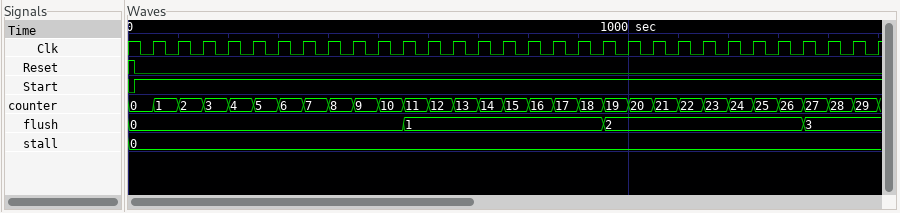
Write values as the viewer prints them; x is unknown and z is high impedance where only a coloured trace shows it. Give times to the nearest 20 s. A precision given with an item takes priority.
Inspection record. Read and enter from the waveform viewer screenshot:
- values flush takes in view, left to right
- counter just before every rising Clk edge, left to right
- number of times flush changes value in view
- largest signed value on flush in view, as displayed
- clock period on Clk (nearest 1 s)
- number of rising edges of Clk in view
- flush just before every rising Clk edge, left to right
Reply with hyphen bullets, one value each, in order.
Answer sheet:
- 0, 1, 2, 3
- 0, 1, 2, 3, 4, 5, 6, 7, 8, 9, 10, 11, 12, 13, 14, 15, 16, 17, 18, 19, 20, 21, 22, 23, 24, 25, 26, 27, 28, 29
- 3
- 3
- 50 s
- 30
- 0, 0, 0, 0, 0, 0, 0, 0, 0, 0, 0, 1, 1, 1, 1, 1, 1, 1, 1, 2, 2, 2, 2, 2, 2, 2, 2, 3, 3, 3
